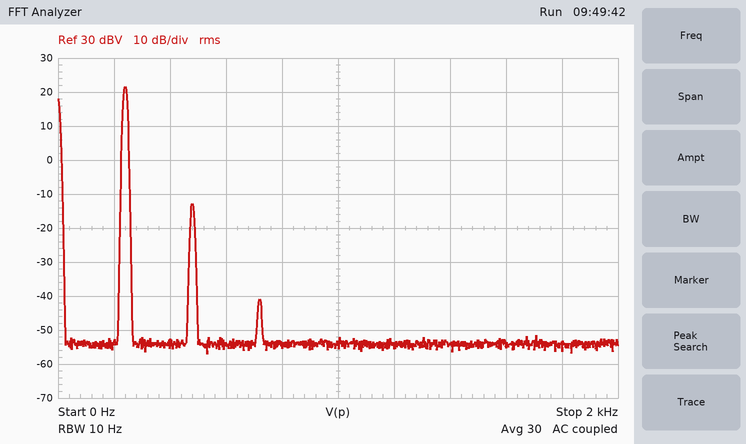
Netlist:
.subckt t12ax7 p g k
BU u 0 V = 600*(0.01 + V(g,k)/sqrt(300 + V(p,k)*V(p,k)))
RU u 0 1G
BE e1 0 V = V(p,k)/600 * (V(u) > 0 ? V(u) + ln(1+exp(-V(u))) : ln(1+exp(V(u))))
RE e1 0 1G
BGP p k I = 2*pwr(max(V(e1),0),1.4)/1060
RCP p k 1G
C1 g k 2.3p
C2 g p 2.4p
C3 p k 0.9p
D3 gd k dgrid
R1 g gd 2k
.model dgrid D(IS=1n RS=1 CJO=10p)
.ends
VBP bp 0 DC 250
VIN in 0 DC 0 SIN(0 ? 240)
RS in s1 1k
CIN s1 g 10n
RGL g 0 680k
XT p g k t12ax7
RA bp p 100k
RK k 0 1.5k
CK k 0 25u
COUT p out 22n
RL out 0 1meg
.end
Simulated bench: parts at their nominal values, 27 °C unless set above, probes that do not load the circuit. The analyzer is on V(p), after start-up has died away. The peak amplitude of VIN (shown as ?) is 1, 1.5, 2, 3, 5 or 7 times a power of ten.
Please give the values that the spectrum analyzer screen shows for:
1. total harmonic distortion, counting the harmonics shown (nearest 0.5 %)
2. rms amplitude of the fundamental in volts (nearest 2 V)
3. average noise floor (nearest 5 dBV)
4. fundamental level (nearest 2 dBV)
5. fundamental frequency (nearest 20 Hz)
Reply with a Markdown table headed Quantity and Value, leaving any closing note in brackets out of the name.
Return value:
| Quantity | Value |
|---|---|
| total harmonic distortion, counting the harmonics shown | 2.0 % |
| rms amplitude of the fundamental in volts | 12 V |
| average noise floor | -55 dBV |
| fundamental level | 22 dBV |
| fundamental frequency | 240 Hz |
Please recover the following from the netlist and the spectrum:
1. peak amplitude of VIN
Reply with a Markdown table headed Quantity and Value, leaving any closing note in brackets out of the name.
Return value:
| Quantity | Value |
|---|---|
| peak amplitude of VIN | 300 mV |
